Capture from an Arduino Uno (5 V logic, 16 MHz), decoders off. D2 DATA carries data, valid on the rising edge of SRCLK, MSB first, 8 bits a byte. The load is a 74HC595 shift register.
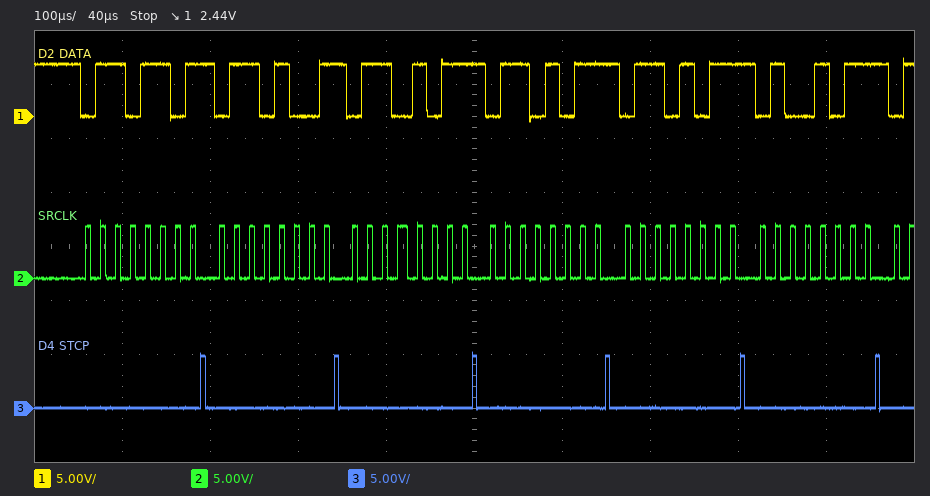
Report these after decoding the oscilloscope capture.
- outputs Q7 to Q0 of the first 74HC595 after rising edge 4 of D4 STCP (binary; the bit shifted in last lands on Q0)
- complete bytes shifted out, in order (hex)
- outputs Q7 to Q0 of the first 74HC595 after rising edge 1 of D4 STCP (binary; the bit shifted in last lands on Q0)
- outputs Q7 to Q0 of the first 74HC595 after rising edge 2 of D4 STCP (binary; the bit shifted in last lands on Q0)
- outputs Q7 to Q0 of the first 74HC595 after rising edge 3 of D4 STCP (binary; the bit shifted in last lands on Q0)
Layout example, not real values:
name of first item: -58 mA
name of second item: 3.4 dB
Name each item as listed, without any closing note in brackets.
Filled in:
outputs Q7 to Q0 of the first 74HC595 after rising edge 4 of D4 STCP: 01101011
complete bytes shifted out, in order: 6D 69 6B 6B 6B 4B
outputs Q7 to Q0 of the first 74HC595 after rising edge 1 of D4 STCP: 01101101
outputs Q7 to Q0 of the first 74HC595 after rising edge 2 of D4 STCP: 01101001
outputs Q7 to Q0 of the first 74HC595 after rising edge 3 of D4 STCP: 01101011
